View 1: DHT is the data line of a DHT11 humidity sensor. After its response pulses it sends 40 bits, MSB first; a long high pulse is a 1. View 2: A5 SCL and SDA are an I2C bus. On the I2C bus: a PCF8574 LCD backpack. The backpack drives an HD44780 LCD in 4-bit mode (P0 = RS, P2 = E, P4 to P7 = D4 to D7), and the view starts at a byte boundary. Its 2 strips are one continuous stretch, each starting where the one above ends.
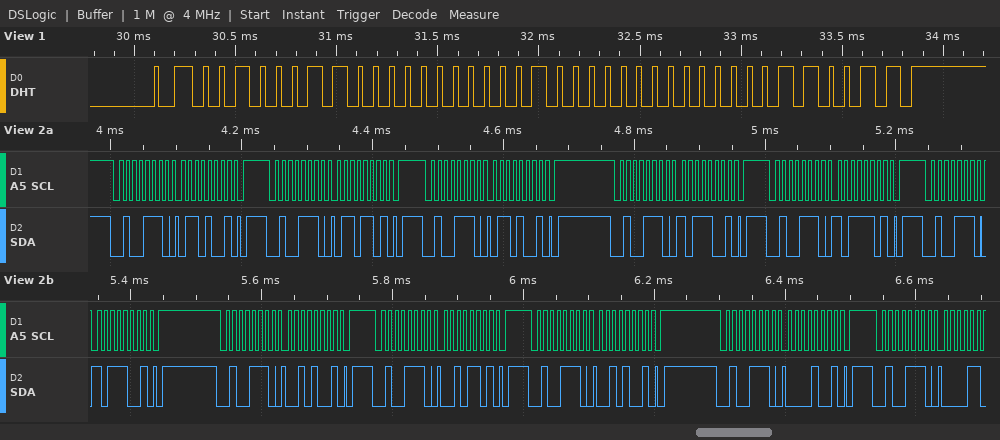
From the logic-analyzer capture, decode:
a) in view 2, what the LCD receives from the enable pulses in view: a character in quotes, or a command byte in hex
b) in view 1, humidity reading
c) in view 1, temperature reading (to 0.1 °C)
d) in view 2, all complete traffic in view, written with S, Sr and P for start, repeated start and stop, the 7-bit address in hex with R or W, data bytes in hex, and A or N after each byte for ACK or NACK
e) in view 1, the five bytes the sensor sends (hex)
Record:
'k'
35 %
16.0 °C
S 27W A 69 A P S 27W A 6D A P S 27W A 69 A P S 27W A B9 A P S 27W A BD A P S 27W A B9 A P S 27W A 29 A P S 27W A 2D A P S 27W A 29 A P S 27W A 09 A P S 27W A
23 00 10 00 33
